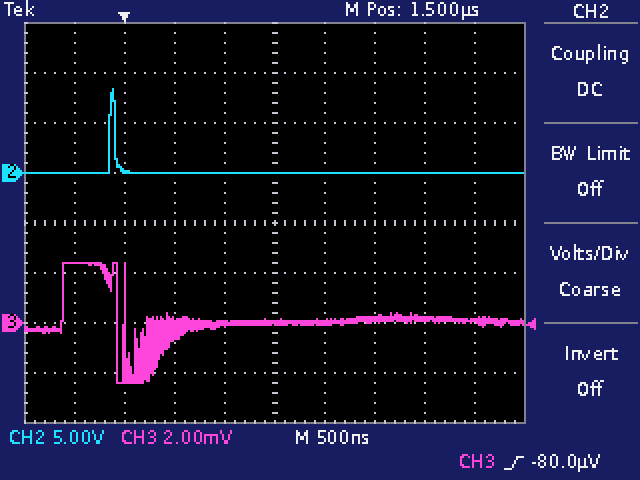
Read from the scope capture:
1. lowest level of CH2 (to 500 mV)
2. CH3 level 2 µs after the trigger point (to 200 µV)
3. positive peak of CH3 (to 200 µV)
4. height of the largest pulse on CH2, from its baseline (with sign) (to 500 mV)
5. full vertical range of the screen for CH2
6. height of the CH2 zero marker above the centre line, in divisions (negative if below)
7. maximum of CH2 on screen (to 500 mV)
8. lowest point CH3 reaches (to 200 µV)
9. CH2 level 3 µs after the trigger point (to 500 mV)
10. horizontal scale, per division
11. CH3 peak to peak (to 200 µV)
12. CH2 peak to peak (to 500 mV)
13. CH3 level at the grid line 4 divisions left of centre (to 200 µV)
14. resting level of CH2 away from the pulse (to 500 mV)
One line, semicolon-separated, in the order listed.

0.0 V; 0.0 mV; 2.4 mV; +8.5 V; 40 V; +1.0 div; 8.5 V; -2.4 mV; 0.0 V; 500 ns; 4.8 mV; 8.5 V; 2.4 mV; 0.0 V
